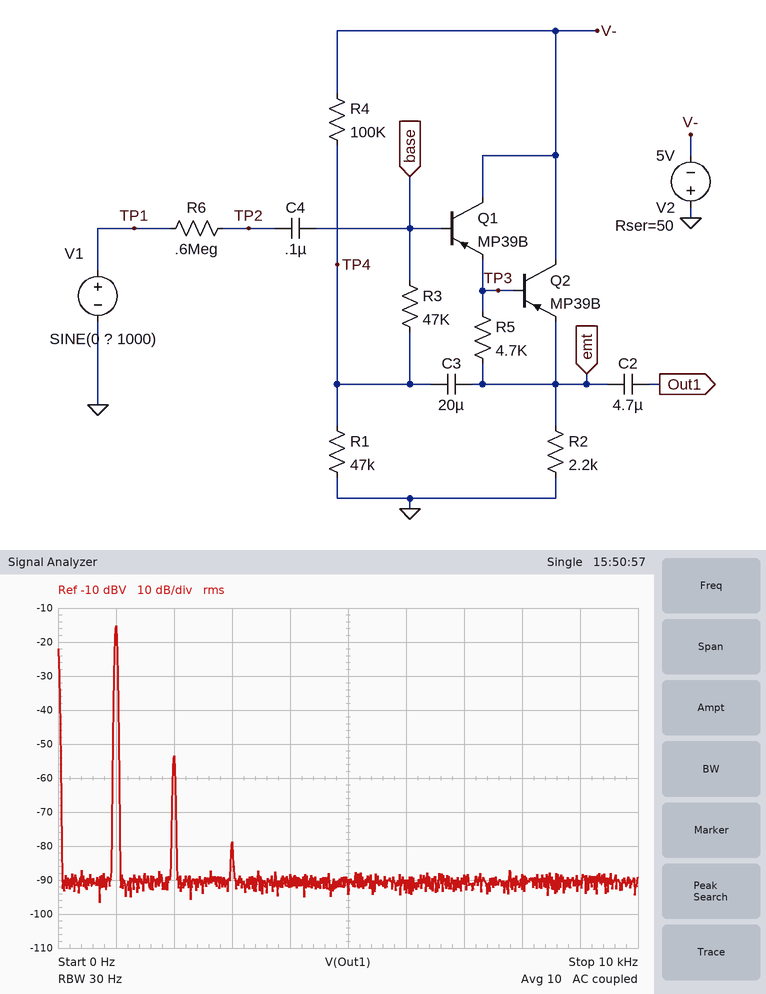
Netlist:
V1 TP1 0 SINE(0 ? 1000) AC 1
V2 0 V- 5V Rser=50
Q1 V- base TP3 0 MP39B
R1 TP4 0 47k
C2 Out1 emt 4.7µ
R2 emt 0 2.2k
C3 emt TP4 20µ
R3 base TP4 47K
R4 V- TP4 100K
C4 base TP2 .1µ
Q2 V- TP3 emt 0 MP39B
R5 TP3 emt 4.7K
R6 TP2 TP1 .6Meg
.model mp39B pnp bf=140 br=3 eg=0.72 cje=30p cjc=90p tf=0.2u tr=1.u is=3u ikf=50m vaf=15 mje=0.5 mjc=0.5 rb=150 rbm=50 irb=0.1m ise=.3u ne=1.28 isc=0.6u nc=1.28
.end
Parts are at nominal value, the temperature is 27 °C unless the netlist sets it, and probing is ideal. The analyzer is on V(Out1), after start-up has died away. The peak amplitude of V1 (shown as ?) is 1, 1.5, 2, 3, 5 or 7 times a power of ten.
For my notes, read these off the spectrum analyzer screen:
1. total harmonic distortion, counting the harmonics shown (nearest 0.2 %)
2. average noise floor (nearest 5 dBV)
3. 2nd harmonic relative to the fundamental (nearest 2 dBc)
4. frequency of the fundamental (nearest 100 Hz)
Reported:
1.2 %
-90 dBV
-38 dBc
1.0 kHz
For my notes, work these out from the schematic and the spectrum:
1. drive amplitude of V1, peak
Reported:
500 mV
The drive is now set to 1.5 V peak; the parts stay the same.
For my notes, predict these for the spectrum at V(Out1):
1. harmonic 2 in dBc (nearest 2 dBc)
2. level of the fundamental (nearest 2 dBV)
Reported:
-28 dBc
-6 dBV
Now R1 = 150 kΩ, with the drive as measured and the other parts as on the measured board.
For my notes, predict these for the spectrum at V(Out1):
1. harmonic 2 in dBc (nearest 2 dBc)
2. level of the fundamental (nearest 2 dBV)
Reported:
-50 dBc
-14 dBV
